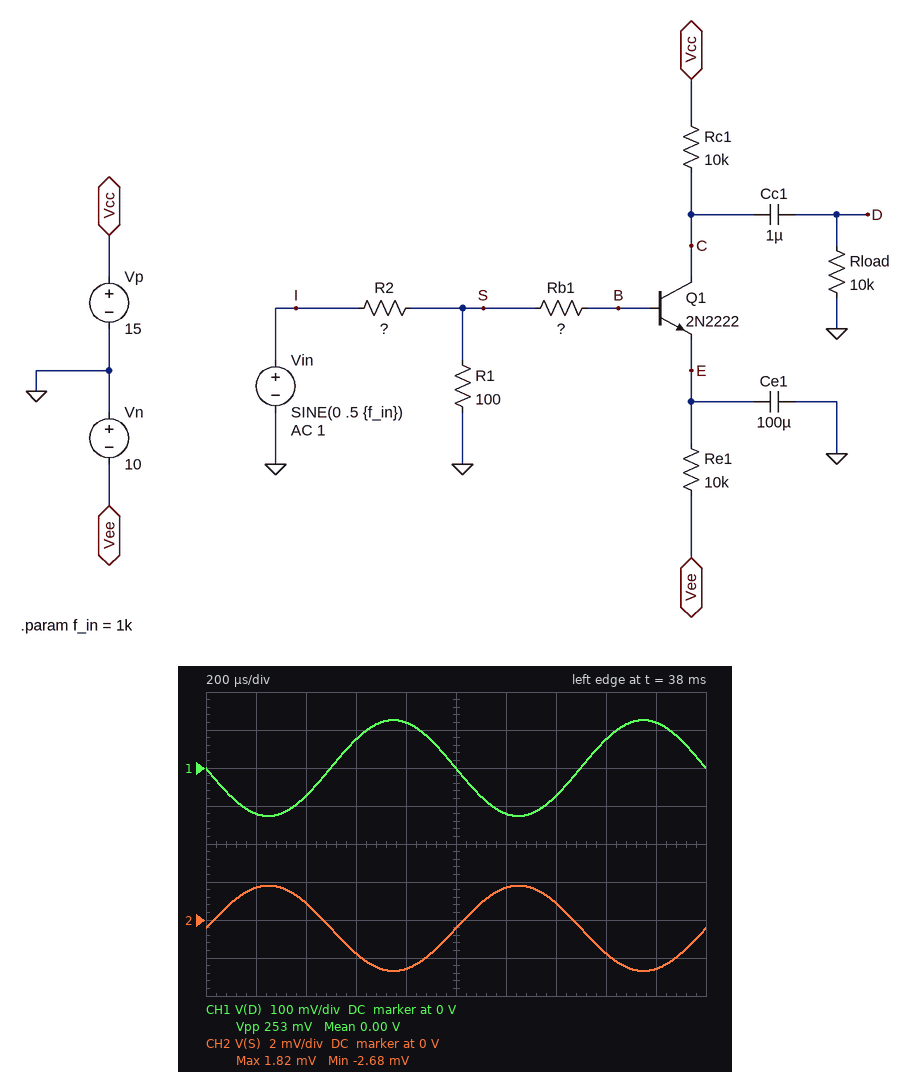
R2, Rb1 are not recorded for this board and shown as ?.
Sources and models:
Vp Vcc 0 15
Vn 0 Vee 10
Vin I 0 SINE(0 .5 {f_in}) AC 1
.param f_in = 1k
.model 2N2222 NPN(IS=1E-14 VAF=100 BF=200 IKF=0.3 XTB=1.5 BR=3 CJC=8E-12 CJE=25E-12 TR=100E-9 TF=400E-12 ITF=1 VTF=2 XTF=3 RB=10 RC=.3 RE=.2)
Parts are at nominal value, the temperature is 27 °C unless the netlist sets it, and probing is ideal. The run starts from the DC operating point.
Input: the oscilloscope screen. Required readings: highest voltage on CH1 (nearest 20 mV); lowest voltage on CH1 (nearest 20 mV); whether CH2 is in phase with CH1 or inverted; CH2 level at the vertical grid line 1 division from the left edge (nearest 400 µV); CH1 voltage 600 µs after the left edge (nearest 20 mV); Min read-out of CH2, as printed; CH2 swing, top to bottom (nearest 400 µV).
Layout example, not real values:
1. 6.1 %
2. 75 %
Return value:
1. 120 mV
2. -120 mV
3. inverted
4. 1.6 mV
5. 80 mV
6. -2.68 mV
7. 4.4 mV
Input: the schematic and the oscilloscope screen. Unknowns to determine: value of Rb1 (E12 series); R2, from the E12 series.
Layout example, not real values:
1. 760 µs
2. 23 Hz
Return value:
1. 12 kΩ
2. 22 kΩ
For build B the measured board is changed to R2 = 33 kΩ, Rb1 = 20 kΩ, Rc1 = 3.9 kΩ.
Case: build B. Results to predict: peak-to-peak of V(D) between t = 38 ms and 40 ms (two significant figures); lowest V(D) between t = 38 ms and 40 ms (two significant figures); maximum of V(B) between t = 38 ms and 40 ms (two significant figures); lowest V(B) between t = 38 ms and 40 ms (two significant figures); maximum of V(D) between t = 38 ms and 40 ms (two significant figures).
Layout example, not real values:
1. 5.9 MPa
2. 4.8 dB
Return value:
1. 70 mV
2. -35 mV
3. -83 mV
4. -84 mV
5. 35 mV
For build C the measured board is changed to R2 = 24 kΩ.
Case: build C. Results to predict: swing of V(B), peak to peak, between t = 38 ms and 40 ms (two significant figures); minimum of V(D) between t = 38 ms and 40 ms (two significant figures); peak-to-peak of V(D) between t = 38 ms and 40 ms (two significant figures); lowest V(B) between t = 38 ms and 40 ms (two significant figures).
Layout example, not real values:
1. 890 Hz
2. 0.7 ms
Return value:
1. 1.4 mV
2. -120 mV
3. 230 mV
4. -54 mV
